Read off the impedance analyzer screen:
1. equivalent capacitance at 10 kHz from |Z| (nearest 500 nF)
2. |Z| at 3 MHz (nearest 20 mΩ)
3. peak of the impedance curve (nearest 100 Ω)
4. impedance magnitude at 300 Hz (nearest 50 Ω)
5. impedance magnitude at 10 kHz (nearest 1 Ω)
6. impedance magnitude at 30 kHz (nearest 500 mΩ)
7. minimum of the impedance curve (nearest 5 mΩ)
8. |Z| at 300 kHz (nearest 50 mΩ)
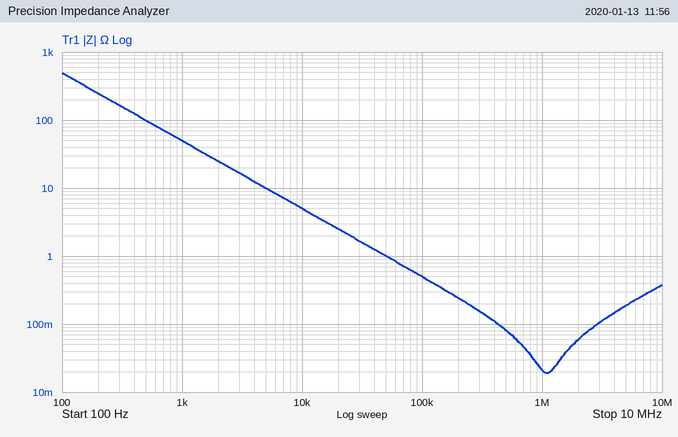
3.0 µF
100 mΩ
500 Ω
150 Ω
5 Ω
1.5 Ω
20 mΩ
150 mΩ
